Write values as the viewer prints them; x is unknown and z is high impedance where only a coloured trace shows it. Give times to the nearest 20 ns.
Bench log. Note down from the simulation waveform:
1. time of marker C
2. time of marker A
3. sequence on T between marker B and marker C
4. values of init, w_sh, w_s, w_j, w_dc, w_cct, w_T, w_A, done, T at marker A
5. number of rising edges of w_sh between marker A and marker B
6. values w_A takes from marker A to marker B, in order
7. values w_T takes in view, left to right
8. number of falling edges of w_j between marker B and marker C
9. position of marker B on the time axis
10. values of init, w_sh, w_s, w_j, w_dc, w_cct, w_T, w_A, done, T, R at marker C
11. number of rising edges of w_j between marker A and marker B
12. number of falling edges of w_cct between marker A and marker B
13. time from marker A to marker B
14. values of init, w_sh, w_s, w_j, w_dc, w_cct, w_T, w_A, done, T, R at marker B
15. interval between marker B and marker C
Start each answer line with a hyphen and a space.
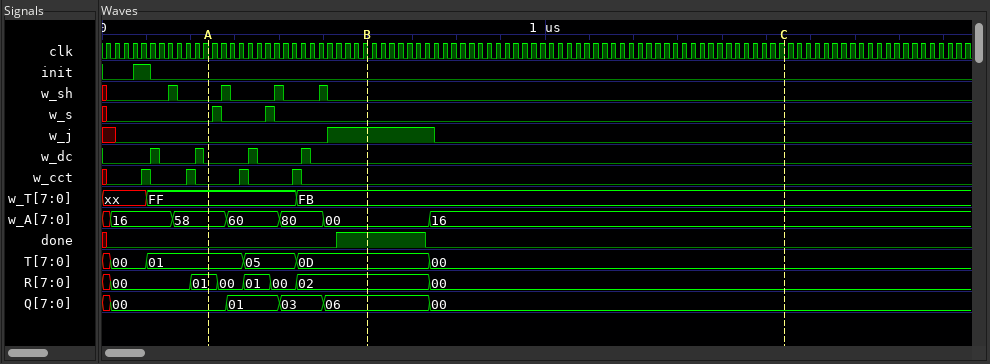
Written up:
- 1540 ns
- 240 ns
- 0D, 00
- init=0, w_sh=0, w_s=0, w_j=0, w_dc=0, w_cct=0, w_T=FF, w_A=58, done=0, T=01
- 3
- 58, 60, 80, 00
- xx, FF, FB
- 1
- 600 ns
- init=0, w_sh=0, w_s=0, w_j=0, w_dc=0, w_cct=0, w_T=FB, w_A=16, done=0, T=00, R=00
- 1
- 2
- 360 ns
- init=0, w_sh=0, w_s=0, w_j=1, w_dc=0, w_cct=0, w_T=FB, w_A=00, done=1, T=0D, R=02
- 940 ns
